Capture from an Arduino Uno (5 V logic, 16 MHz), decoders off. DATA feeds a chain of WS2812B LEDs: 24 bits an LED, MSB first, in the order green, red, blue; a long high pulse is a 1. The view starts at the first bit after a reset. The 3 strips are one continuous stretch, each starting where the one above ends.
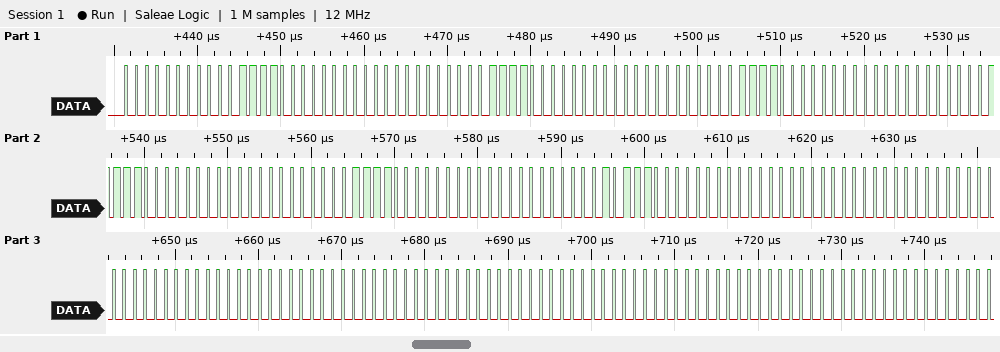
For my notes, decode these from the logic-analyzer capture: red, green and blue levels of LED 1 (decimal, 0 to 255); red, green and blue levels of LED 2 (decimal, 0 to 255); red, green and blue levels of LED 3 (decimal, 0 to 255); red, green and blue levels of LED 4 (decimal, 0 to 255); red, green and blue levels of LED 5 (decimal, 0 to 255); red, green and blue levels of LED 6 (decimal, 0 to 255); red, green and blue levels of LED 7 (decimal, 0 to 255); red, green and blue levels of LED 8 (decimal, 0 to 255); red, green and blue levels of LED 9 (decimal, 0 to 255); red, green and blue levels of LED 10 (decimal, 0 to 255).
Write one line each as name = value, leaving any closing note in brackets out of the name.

red, green and blue levels of LED 1 = 30, 0, 0
red, green and blue levels of LED 2 = 30, 0, 0
red, green and blue levels of LED 3 = 30, 0, 0
red, green and blue levels of LED 4 = 30, 0, 0
red, green and blue levels of LED 5 = 30, 0, 0
red, green and blue levels of LED 6 = 23, 0, 0
red, green and blue levels of LED 7 = 0, 0, 0
red, green and blue levels of LED 8 = 0, 0, 0
red, green and blue levels of LED 9 = 0, 0, 0
red, green and blue levels of LED 10 = 0, 0, 0
